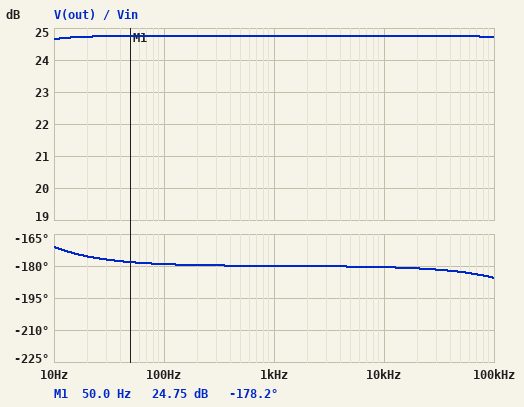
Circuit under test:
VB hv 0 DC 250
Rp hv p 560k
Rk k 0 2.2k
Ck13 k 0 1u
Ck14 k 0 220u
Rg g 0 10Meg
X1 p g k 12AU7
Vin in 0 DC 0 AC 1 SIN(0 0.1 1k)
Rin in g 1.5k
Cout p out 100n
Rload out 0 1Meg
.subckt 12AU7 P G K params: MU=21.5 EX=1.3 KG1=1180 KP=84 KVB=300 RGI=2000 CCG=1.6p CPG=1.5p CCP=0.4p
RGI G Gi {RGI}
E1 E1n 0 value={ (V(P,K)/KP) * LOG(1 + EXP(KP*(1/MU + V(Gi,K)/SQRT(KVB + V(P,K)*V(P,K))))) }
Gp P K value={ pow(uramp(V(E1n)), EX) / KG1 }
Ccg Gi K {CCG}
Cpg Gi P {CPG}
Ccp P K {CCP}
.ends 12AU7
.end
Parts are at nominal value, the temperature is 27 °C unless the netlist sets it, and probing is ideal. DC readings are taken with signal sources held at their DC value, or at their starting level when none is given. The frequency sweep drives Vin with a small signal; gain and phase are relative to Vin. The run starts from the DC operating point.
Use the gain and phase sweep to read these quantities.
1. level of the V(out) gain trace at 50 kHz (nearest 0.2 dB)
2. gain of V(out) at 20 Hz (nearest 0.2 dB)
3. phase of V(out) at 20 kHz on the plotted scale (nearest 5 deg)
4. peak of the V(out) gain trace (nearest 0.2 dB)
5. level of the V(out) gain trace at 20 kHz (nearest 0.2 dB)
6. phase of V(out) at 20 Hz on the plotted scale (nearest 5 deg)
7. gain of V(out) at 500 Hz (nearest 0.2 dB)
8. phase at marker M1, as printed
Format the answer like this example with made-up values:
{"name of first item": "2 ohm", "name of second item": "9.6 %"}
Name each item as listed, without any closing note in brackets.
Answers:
{"level of the V(out) gain trace at 50 kHz": "24.8 dB", "gain of V(out) at 20 Hz": "24.8 dB", "phase of V(out) at 20 kHz on the plotted scale": "-180 deg", "peak of the V(out) gain trace": "24.8 dB", "level of the V(out) gain trace at 20 kHz": "24.8 dB", "phase of V(out) at 20 Hz on the plotted scale": "-175 deg", "gain of V(out) at 500 Hz": "24.8 dB", "phase at marker M1, as printed": "-178.2 deg"}
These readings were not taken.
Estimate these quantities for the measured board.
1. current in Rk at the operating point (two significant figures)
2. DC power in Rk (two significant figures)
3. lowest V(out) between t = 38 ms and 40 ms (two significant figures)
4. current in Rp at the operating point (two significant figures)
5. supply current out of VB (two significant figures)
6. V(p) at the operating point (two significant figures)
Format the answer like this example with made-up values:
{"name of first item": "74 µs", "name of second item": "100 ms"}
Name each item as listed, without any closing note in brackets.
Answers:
{"current in Rk at the operating point": "400 µA", "DC power in Rk": "350 µW", "lowest V(out) between t = 38 ms and 40 ms": "-1.7 V", "current in Rp at the operating point": "400 µA", "supply current out of VB": "400 µA", "V(p) at the operating point": "27 V"}
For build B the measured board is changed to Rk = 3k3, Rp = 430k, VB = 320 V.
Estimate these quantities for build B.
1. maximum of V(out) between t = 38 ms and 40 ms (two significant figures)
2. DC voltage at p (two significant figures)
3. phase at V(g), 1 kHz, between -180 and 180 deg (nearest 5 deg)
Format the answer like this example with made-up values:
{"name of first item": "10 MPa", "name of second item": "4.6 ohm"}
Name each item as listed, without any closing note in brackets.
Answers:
{"maximum of V(out) between t = 38 ms and 40 ms": "1.6 V", "DC voltage at p": "56 V", "phase at V(g), 1 kHz, between -180 and 180 deg": "0 deg"}
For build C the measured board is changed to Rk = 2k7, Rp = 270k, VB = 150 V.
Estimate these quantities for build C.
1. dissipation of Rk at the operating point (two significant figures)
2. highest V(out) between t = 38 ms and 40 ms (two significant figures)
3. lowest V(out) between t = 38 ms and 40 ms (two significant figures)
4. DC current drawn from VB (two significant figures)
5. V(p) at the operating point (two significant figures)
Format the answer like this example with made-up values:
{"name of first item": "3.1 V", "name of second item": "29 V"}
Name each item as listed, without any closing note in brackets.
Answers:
{"dissipation of Rk at the operating point": "500 µW", "highest V(out) between t = 38 ms and 40 ms": "1.6 V", "lowest V(out) between t = 38 ms and 40 ms": "-1.6 V", "DC current drawn from VB": "430 µA", "V(p) at the operating point": "34 V"}
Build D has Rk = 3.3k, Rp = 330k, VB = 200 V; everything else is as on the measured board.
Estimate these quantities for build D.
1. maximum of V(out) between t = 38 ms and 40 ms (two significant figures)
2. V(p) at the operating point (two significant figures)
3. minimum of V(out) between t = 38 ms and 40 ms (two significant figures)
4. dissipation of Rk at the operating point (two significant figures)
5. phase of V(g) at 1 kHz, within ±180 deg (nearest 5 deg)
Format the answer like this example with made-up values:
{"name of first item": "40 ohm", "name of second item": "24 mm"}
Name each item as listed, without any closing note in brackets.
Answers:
{"maximum of V(out) between t = 38 ms and 40 ms": "1.6 V", "V(p) at the operating point": "43 V", "minimum of V(out) between t = 38 ms and 40 ms": "-1.6 V", "dissipation of Rk at the operating point": "750 µW", "phase of V(g) at 1 kHz, within ±180 deg": "0 deg"}
